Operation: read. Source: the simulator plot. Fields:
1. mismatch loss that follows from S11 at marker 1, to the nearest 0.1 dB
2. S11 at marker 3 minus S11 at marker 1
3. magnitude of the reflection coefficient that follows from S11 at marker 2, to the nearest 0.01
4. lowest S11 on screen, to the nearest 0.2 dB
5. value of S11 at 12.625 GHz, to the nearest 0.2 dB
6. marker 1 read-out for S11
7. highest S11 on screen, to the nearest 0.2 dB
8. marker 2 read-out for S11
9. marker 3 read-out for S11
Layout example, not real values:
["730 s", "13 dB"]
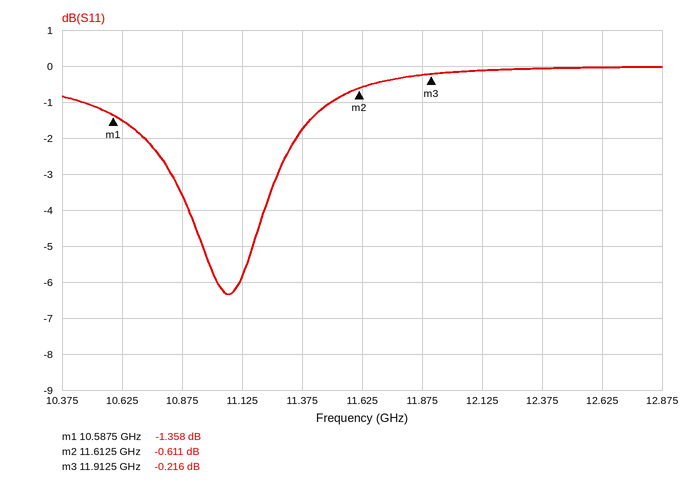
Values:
["5.7 dB", "1.142 dB", "0.93", "-6.4 dB", "0.0 dB", "-1.358 dB", "0.0 dB", "-0.611 dB", "-0.216 dB"]
